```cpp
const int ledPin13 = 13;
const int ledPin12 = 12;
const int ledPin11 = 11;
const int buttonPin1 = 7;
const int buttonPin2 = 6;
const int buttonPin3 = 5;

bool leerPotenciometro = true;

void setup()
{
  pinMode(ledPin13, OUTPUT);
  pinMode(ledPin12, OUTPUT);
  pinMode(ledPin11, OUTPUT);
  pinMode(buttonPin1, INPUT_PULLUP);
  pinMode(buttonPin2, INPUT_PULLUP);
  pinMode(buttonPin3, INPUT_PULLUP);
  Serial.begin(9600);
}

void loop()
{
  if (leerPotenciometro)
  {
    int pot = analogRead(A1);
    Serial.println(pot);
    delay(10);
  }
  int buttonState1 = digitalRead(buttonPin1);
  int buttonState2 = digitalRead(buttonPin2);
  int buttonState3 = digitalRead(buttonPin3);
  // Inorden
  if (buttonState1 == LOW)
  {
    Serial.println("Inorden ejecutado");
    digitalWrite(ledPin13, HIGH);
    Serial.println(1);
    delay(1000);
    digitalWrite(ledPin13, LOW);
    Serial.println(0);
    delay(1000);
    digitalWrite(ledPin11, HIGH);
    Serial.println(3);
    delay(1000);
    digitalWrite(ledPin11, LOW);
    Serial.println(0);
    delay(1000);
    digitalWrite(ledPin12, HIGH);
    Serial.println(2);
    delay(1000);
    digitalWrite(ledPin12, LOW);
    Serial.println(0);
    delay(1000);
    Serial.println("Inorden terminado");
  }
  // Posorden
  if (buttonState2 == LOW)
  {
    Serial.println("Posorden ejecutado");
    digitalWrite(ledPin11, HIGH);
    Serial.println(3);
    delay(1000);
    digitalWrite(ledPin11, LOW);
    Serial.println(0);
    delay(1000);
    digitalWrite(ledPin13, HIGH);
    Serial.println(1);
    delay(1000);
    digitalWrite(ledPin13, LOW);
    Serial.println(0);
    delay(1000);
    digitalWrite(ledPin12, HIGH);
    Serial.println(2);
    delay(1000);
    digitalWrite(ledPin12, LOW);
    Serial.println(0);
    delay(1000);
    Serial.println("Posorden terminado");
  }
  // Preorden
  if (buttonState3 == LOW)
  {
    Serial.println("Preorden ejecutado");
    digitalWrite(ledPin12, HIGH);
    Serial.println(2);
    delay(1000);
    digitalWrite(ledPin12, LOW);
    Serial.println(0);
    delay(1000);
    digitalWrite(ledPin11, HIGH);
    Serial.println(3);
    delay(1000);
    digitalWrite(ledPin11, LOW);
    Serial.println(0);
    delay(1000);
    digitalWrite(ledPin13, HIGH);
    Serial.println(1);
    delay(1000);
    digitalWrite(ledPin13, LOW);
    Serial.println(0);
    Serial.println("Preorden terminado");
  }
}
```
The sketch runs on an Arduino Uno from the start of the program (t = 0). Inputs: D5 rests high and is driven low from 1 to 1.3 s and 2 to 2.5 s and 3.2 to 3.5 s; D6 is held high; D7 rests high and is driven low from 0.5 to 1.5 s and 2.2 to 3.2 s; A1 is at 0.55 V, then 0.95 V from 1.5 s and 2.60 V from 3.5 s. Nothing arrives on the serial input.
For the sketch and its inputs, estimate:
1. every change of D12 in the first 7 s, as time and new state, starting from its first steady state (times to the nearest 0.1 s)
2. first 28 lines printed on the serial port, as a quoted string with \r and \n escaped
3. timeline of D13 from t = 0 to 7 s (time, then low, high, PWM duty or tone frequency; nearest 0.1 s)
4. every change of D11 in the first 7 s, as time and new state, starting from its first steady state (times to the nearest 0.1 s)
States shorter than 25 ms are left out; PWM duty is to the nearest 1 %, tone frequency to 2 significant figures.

0 s low; 4.5 s high; 5.5 s low
"112\r\n112\r\n112\r\n112\r\n112\r\n112\r\n112\r\n112\r\n112\r\n112\r\n112\r\n112\r\n112\r\n112\r\n112\r\n112\r\n112\r\n112\r\n112\r\n112\r\n112\r\n112\r\n112\r\n112\r\n112\r\n112\r\n112\r\n112\r\n"
0 s low; 0.5 s high; 1.5 s low
0 s low; 2.5 s high; 3.5 s low
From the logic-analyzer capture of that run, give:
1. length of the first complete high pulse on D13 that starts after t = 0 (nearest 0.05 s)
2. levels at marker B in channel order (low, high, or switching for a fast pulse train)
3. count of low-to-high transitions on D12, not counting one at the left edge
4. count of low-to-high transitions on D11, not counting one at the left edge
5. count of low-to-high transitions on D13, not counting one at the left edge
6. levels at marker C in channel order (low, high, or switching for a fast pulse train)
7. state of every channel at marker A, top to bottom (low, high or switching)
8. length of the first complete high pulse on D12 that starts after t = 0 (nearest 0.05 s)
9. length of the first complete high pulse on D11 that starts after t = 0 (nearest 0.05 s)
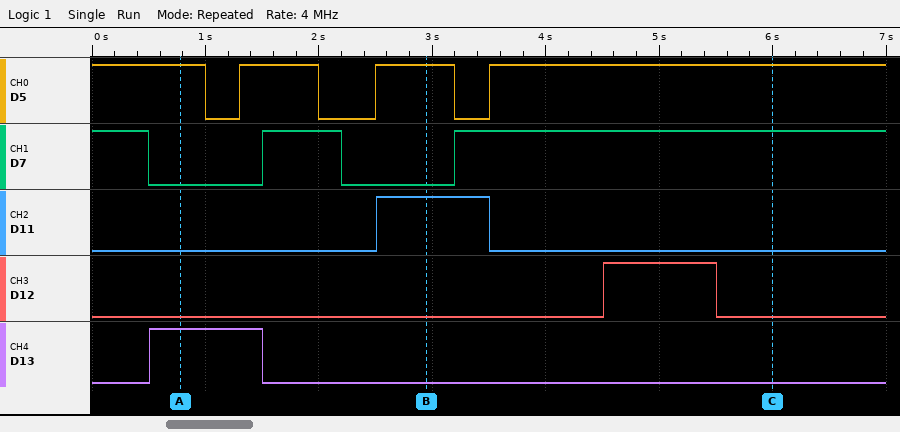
1.00 s
D5 high, D7 low, D11 high, D12 low, D13 low
1
1
1
D5 high, D7 high, D11 low, D12 low, D13 low
D5 high, D7 low, D11 low, D12 low, D13 high
1.00 s
1.00 s
